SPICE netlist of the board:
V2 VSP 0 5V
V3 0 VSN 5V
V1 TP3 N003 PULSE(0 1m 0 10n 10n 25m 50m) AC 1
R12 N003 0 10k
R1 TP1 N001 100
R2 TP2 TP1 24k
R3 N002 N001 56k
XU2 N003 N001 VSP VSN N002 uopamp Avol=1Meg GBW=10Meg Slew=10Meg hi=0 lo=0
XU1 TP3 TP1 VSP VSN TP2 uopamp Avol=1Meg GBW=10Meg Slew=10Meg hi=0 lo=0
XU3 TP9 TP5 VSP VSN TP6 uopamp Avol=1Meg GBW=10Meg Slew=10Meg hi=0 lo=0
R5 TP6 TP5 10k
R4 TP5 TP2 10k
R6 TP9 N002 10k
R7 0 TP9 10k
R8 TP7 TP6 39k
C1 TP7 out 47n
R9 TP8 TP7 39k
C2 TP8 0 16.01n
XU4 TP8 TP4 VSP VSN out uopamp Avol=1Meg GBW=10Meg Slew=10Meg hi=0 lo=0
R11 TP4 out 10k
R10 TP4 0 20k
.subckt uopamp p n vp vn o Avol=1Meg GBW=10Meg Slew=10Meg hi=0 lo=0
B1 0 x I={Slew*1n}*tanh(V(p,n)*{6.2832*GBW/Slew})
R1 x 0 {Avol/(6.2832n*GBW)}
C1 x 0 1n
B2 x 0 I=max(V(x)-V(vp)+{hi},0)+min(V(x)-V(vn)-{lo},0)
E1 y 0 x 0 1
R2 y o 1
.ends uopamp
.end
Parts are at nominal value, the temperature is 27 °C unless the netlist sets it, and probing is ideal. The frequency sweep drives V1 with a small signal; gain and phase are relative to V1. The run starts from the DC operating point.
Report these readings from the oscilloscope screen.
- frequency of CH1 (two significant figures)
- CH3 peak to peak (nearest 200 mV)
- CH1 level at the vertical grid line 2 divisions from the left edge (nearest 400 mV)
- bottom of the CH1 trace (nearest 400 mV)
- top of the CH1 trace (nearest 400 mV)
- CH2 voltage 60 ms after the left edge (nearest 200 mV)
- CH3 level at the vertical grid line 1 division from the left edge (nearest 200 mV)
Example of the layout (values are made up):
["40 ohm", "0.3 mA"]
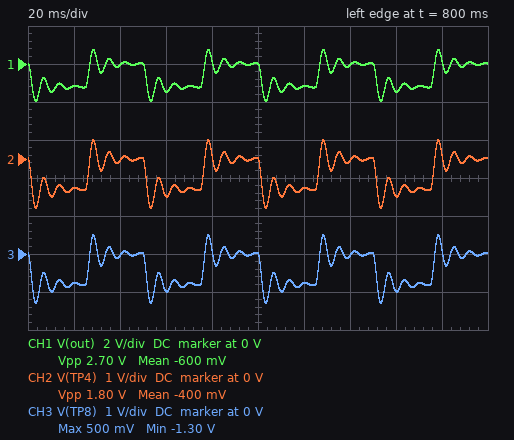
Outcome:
["20 Hz", "1.8 V", "0 V", "-2.0 V", "800 mV", "-1.0 V", "-800 mV"]
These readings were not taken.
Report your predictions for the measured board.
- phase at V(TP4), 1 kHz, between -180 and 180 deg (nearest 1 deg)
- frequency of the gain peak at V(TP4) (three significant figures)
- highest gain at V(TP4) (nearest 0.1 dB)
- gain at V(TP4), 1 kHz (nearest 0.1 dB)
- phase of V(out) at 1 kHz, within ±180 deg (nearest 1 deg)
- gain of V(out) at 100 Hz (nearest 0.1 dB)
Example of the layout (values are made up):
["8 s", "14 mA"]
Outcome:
["-2 deg", "145 Hz", "68.3 dB", "25.1 dB", "-2 deg", "66.2 dB"]
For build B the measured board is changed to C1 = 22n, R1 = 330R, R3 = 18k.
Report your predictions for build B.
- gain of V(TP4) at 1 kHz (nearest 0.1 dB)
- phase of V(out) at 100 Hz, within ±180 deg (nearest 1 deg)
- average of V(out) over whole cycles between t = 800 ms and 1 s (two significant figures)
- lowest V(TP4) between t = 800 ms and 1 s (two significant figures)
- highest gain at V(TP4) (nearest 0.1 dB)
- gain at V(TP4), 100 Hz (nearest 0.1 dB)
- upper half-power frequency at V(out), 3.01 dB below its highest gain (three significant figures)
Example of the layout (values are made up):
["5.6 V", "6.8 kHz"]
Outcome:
["15.8 dB", "147 deg", "-96 mV", "-140 mV", "42.8 dB", "42.7 dB", "248 Hz"]
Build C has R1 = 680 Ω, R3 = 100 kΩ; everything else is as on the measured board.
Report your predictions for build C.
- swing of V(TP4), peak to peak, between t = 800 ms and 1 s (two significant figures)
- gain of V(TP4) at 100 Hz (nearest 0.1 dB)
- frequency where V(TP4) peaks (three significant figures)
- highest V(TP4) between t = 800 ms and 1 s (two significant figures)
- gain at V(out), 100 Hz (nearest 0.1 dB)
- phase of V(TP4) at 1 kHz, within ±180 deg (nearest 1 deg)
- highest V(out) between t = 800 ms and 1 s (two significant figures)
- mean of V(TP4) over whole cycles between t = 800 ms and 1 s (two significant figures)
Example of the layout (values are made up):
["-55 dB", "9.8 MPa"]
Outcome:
["410 mV", "49.9 dB", "145 Hz", "110 mV", "53.4 dB", "2 deg", "170 mV", "-92 mV"]
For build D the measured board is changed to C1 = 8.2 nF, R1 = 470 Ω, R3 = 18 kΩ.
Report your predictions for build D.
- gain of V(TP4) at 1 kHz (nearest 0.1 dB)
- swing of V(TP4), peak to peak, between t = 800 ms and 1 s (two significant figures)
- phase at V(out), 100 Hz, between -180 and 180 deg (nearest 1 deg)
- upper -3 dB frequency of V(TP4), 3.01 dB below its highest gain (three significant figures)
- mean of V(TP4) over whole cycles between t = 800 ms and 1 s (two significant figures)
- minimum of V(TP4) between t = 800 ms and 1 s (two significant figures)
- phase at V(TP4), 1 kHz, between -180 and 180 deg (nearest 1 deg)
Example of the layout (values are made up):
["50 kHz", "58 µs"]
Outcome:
["19.4 dB", "90 mV", "143 deg", "174 Hz", "-45 mV", "-90 mV", "44 deg"]
